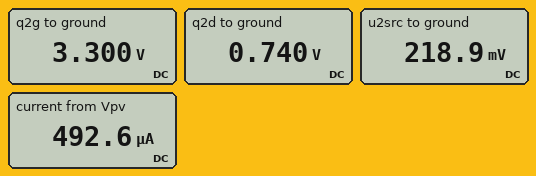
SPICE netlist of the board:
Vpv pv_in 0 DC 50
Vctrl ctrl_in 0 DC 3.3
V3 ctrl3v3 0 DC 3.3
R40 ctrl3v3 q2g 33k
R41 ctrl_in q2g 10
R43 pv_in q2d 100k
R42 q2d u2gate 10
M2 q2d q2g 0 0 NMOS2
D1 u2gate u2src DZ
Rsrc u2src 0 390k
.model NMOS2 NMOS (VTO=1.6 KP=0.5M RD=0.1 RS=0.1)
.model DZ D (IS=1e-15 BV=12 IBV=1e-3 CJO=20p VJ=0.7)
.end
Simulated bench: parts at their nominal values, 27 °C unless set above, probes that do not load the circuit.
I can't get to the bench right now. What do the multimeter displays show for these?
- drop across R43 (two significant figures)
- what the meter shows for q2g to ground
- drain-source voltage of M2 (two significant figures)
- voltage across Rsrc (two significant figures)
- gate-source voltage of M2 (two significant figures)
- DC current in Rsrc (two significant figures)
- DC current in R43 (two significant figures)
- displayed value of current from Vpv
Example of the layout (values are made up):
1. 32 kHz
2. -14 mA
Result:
1. 49 V
2. 3.300 V
3. 740 mV
4. 220 mV
5. 3.3 V
6. 560 nA
7. 490 µA
8. 492.6 µA
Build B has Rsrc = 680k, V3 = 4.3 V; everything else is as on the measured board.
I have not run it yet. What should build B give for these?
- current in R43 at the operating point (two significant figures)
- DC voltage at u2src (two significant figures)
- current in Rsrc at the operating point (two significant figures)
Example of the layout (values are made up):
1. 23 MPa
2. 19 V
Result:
1. 490 µA
2. 230 mV
3. 340 nA
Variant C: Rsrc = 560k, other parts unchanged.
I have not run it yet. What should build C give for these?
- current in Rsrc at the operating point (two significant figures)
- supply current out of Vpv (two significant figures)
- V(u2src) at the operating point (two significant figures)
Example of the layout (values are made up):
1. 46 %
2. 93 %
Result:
1. 410 nA
2. 490 µA
3. 230 mV
